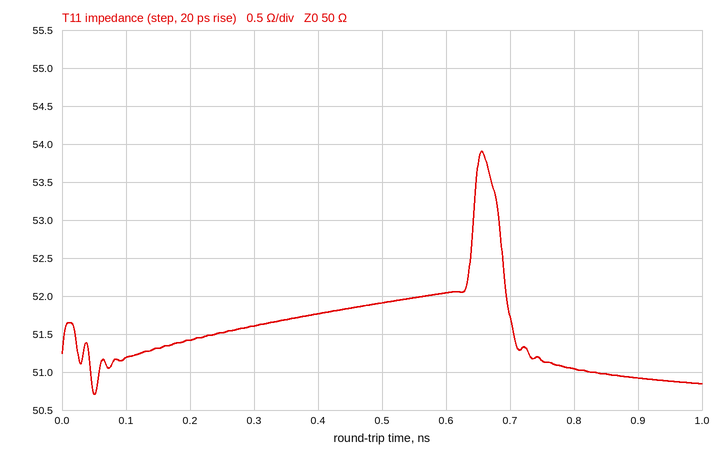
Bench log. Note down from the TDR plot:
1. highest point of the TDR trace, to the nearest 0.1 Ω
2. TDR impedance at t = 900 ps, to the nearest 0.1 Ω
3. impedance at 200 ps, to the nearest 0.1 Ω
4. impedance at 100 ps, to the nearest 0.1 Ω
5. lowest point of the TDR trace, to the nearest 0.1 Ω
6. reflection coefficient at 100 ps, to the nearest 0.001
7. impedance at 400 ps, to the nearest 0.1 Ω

53.9 Ω
50.9 Ω
51.4 Ω
51.2 Ω
50.7 Ω
+0.012
51.8 Ω
